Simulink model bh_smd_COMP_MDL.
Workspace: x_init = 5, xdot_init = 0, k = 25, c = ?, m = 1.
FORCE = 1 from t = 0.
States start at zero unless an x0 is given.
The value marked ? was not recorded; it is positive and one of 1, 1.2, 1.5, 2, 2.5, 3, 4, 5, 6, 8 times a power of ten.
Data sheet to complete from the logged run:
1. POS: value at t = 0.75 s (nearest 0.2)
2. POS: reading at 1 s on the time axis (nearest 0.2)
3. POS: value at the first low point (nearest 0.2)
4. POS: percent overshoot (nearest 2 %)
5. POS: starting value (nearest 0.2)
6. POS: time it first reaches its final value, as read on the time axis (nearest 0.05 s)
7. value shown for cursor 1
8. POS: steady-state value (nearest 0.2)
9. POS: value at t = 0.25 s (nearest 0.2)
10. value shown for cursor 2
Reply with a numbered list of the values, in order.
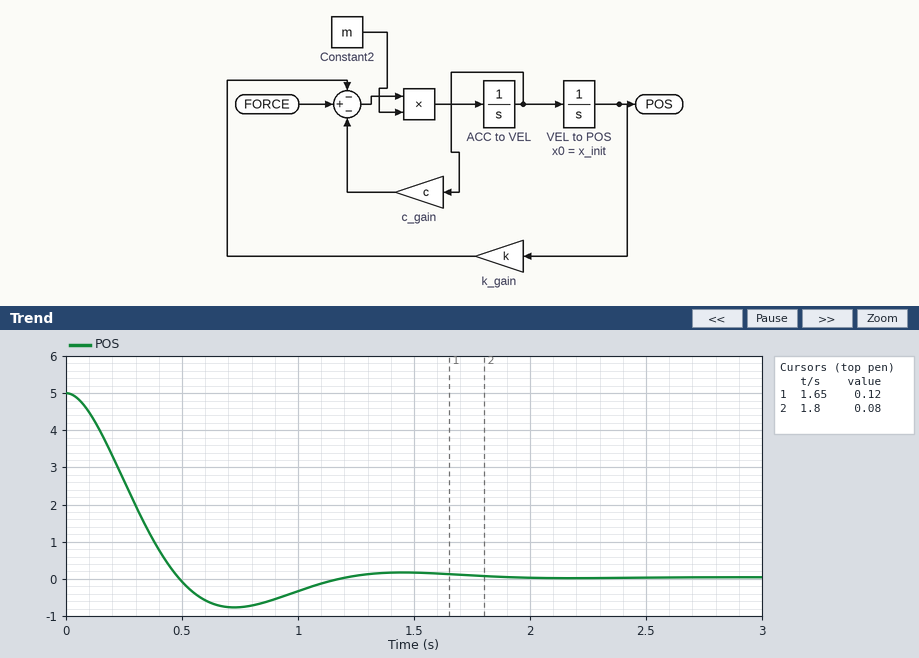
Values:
1. -0.8
2. -0.4
3. -0.8
4. 16 %
5. 5.0
6. 0.50 s
7. 0.12
8. 0.0
9. 2.6
10. 0.08
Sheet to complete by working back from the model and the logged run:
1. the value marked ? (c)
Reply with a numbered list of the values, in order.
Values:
1. 5
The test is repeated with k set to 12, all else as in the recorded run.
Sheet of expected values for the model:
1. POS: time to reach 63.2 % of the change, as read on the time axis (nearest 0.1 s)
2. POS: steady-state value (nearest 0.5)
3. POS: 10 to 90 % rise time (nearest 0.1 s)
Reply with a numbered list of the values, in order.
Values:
1. 0.5 s
2. 0.0
3. 0.6 s
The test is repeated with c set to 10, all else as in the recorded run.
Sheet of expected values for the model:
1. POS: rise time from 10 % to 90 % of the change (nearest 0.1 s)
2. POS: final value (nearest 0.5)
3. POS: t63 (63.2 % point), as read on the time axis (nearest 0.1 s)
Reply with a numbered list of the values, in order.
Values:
1. 0.7 s
2. 0.0
3. 0.4 s
